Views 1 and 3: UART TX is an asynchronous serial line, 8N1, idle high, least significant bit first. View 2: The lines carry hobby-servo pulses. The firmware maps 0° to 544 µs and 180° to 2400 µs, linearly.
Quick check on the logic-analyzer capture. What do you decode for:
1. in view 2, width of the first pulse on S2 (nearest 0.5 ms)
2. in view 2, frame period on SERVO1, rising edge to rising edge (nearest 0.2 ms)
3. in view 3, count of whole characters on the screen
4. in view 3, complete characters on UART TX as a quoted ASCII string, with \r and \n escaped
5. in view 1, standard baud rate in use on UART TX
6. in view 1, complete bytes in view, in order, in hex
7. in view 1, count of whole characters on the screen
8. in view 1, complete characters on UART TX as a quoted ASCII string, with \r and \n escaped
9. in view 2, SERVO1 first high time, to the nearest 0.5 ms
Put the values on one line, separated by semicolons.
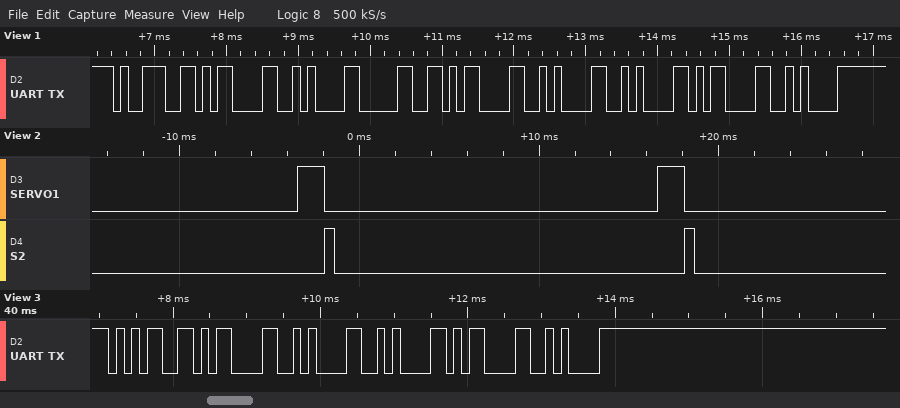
0.5 ms; 20.0 ms; 6; "5\r\n\n\r\n"; 9600 baud; 0x39 0x0D 0x0A 0x30 0x0D 0x0A 0x0A 0x0D 0x0A; 9; "9\r\n0\r\n\n\r\n"; 1.5 ms
